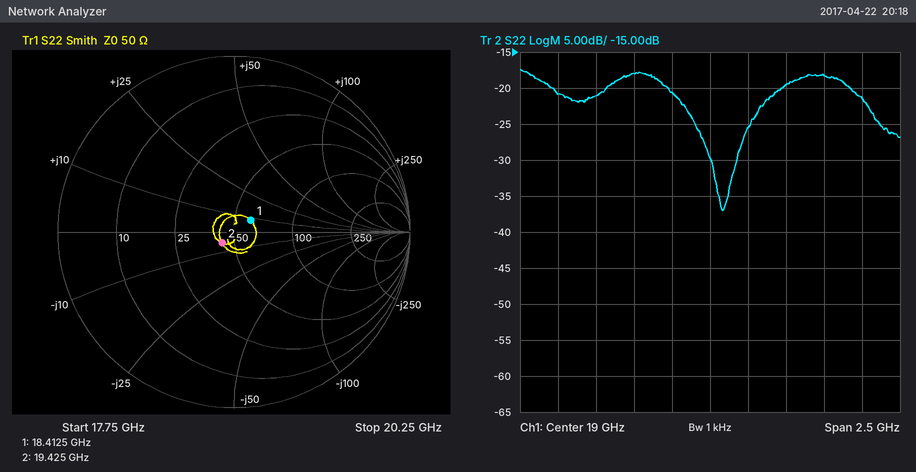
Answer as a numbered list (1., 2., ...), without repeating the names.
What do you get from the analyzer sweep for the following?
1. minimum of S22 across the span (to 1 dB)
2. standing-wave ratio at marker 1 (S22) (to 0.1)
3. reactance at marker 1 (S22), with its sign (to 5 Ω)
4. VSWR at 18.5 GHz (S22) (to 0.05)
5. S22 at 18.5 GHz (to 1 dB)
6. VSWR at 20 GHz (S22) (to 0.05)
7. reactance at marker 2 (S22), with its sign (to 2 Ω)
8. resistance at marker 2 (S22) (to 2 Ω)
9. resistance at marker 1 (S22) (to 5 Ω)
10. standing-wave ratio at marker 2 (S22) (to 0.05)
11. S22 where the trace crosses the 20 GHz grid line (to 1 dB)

1. -37 dB
2. 1.3
3. +10 Ω
4. 1.30
5. -18 dB
6. 1.20
7. -6 Ω
8. 44 Ω
9. 60 Ω
10. 1.20
11. -21 dB
